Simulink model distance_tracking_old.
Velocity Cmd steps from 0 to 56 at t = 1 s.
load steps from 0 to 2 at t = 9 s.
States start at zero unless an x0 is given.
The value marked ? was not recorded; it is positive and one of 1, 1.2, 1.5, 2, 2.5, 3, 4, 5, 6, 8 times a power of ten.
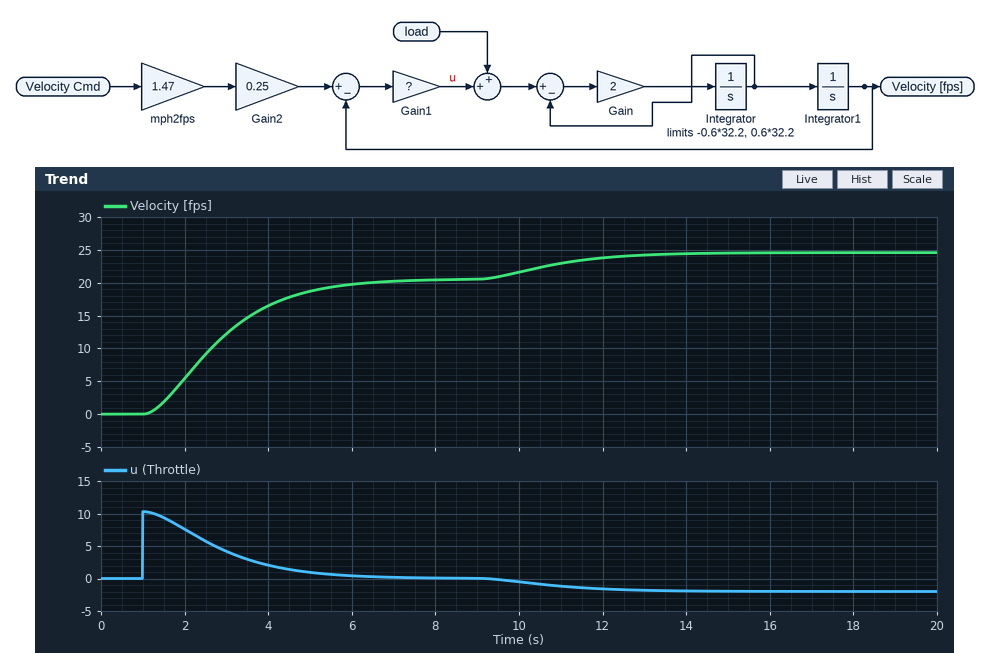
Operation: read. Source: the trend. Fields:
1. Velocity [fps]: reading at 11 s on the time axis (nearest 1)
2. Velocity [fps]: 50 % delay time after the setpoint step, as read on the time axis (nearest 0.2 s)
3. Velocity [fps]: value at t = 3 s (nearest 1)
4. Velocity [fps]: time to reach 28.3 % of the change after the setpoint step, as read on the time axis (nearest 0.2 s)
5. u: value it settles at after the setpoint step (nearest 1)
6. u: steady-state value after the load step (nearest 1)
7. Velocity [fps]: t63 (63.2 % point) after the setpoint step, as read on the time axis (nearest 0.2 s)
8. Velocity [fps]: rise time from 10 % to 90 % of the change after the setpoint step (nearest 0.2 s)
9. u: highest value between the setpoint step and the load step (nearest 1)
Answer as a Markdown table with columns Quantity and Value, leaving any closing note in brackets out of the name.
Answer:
| Quantity | Value |
|---|---|
| Velocity [fps]: reading at 11 s on the time axis | 23 |
| Velocity [fps]: 50 % delay time after the setpoint step, as read on the time axis | 2.6 s |
| Velocity [fps]: value at t = 3 s | 12 |
| Velocity [fps]: time to reach 28.3 % of the change after the setpoint step, as read on the time axis | 2.0 s |
| u: value it settles at after the setpoint step | 0 |
| u: steady-state value after the load step | -2 |
| Velocity [fps]: t63 (63.2 % point) after the setpoint step, as read on the time axis | 3.2 s |
| Velocity [fps]: rise time from 10 % to 90 % of the change after the setpoint step | 3.4 s |
| u: highest value between the setpoint step and the load step | 10 |
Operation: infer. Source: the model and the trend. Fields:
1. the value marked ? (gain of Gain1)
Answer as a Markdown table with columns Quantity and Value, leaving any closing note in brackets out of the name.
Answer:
| Quantity | Value |
|---|---|
| the value marked ? | 0.5 |
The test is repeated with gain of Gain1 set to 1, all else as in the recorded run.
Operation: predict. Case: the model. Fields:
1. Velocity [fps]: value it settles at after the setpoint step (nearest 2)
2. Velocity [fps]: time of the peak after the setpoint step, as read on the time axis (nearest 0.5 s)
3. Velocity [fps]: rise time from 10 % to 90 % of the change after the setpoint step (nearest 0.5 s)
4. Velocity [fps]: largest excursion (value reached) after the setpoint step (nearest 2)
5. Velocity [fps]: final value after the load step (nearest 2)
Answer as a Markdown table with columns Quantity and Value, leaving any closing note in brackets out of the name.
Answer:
| Quantity | Value |
|---|---|
| Velocity [fps]: value it settles at after the setpoint step | 20 |
| Velocity [fps]: time of the peak after the setpoint step, as read on the time axis | 4.0 s |
| Velocity [fps]: rise time from 10 % to 90 % of the change after the setpoint step | 1.5 s |
| Velocity [fps]: largest excursion (value reached) after the setpoint step | 22 |
| Velocity [fps]: final value after the load step | 22 |
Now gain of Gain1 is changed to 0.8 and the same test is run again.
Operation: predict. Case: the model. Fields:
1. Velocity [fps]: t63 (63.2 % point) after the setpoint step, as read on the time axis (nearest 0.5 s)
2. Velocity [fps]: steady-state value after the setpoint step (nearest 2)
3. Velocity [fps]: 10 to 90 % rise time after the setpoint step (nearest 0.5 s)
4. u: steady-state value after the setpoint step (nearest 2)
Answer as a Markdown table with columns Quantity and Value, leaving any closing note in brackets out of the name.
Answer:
| Quantity | Value |
|---|---|
| Velocity [fps]: t63 (63.2 % point) after the setpoint step, as read on the time axis | 2.5 s |
| Velocity [fps]: steady-state value after the setpoint step | 20 |
| Velocity [fps]: 10 to 90 % rise time after the setpoint step | 2.0 s |
| u: steady-state value after the setpoint step | 0 |
